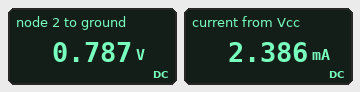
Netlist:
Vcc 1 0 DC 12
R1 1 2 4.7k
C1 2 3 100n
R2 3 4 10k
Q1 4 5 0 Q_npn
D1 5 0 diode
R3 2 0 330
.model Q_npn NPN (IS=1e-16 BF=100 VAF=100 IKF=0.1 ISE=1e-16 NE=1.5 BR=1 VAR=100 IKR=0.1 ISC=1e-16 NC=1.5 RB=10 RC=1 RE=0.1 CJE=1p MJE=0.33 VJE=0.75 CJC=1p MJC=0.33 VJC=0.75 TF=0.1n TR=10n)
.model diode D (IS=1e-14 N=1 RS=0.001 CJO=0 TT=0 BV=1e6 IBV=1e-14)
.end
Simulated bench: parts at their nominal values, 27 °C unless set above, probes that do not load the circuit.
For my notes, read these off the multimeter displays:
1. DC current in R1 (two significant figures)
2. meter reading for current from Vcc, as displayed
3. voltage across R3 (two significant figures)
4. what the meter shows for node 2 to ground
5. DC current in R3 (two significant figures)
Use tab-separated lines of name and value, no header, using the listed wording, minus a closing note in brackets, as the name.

DC current in R1	2.4 mA
meter reading for current from Vcc, as displayed	2.386 mA
voltage across R3	790 mV
what the meter shows for node 2 to ground	0.787 V
DC current in R3	2.4 mA
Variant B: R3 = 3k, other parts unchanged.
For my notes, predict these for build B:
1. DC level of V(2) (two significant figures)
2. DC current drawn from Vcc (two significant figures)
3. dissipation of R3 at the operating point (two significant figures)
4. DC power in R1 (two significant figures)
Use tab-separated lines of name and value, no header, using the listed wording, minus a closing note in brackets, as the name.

DC level of V(2)	4.7 V
DC current drawn from Vcc	1.6 mA
dissipation of R3 at the operating point	7.3 mW
DC power in R1	11 mW
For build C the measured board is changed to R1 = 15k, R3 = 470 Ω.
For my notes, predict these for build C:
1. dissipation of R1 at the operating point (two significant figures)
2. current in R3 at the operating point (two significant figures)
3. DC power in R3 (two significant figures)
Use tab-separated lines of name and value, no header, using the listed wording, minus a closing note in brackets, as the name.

dissipation of R1 at the operating point	9.0 mW
current in R3 at the operating point	780 µA
DC power in R3	280 µW
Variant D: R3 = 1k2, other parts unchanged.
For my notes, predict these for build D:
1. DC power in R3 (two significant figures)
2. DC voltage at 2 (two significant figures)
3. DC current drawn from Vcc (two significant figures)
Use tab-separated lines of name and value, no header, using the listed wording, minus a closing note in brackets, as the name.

DC power in R3	5.0 mW
DC voltage at 2	2.4 V
DC current drawn from Vcc	2.0 mA
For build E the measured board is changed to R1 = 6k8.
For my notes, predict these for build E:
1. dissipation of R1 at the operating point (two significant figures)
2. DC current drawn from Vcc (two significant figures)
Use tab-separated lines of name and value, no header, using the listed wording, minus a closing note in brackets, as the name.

dissipation of R1 at the operating point	19 mW
DC current drawn from Vcc	1.7 mA
